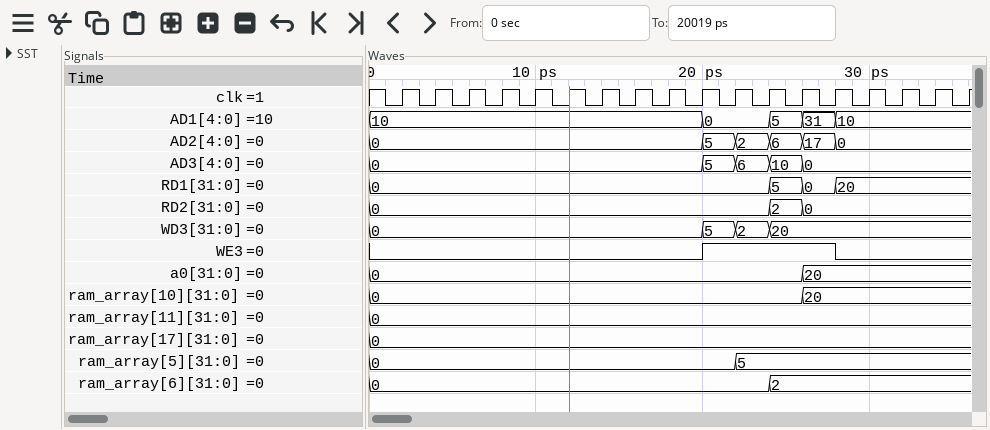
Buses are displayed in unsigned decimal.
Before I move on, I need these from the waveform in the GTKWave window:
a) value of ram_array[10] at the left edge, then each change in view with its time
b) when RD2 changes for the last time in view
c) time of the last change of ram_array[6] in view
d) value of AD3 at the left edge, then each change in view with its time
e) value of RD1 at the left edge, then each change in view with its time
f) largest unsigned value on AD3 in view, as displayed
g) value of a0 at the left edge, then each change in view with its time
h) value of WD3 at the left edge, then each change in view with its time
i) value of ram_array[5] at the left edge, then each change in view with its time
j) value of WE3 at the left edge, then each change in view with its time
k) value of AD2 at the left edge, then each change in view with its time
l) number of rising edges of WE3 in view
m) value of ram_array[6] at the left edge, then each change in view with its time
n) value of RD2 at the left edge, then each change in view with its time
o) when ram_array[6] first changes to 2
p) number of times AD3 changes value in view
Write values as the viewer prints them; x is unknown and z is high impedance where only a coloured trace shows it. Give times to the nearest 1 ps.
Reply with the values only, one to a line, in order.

0, 20 at 26 ps
26 ps
24 ps
0, 5 at 20 ps, 6 at 22 ps, 10 at 24 ps, 0 at 26 ps
0, 5 at 24 ps, 0 at 26 ps, 20 at 28 ps
10
0, 20 at 26 ps
0, 5 at 20 ps, 2 at 22 ps, 20 at 24 ps
0, 5 at 22 ps
0, 1 at 20 ps, 0 at 28 ps
0, 5 at 20 ps, 2 at 22 ps, 6 at 24 ps, 17 at 26 ps, 0 at 28 ps
1
0, 2 at 24 ps
0, 2 at 24 ps, 0 at 26 ps
24 ps
4
